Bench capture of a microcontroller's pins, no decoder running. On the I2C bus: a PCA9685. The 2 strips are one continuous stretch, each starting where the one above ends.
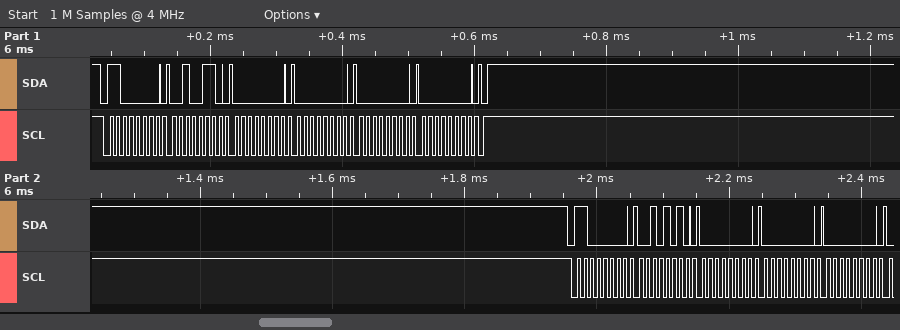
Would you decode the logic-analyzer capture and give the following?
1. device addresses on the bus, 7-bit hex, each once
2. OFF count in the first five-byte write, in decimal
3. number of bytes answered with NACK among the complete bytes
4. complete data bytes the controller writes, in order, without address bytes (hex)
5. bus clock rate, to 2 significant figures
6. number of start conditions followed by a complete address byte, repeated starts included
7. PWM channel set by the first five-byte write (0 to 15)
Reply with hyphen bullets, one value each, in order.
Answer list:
- 0x60
- 0
- 0
- 26 00 00 00 00 2A 00 00 00
- 100 kHz
- 2
- 8
